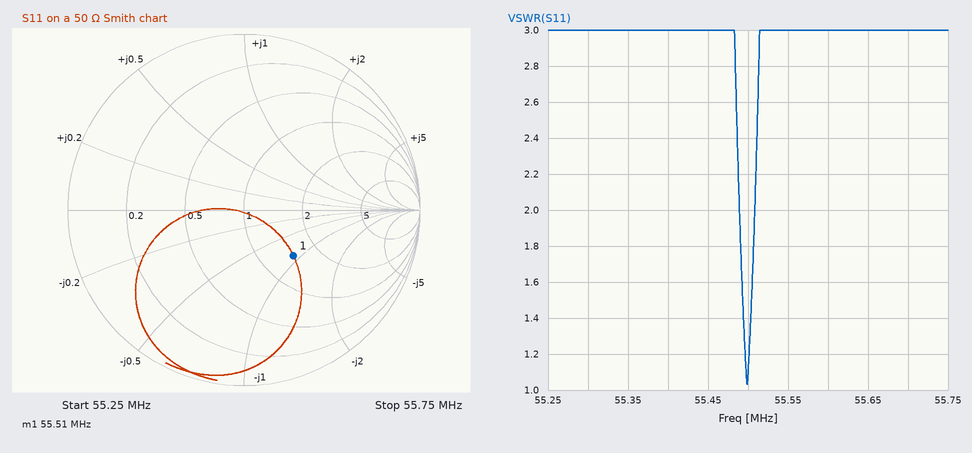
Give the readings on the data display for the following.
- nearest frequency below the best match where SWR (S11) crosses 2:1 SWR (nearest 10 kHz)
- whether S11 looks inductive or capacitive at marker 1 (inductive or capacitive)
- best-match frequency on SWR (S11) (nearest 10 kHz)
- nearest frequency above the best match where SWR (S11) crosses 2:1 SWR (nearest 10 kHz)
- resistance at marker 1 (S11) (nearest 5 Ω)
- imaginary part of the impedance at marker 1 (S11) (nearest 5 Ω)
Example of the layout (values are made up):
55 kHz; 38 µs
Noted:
55.49 MHz; capacitive; 55.50 MHz; 55.51 MHz; 75 Ω; -45 Ω
